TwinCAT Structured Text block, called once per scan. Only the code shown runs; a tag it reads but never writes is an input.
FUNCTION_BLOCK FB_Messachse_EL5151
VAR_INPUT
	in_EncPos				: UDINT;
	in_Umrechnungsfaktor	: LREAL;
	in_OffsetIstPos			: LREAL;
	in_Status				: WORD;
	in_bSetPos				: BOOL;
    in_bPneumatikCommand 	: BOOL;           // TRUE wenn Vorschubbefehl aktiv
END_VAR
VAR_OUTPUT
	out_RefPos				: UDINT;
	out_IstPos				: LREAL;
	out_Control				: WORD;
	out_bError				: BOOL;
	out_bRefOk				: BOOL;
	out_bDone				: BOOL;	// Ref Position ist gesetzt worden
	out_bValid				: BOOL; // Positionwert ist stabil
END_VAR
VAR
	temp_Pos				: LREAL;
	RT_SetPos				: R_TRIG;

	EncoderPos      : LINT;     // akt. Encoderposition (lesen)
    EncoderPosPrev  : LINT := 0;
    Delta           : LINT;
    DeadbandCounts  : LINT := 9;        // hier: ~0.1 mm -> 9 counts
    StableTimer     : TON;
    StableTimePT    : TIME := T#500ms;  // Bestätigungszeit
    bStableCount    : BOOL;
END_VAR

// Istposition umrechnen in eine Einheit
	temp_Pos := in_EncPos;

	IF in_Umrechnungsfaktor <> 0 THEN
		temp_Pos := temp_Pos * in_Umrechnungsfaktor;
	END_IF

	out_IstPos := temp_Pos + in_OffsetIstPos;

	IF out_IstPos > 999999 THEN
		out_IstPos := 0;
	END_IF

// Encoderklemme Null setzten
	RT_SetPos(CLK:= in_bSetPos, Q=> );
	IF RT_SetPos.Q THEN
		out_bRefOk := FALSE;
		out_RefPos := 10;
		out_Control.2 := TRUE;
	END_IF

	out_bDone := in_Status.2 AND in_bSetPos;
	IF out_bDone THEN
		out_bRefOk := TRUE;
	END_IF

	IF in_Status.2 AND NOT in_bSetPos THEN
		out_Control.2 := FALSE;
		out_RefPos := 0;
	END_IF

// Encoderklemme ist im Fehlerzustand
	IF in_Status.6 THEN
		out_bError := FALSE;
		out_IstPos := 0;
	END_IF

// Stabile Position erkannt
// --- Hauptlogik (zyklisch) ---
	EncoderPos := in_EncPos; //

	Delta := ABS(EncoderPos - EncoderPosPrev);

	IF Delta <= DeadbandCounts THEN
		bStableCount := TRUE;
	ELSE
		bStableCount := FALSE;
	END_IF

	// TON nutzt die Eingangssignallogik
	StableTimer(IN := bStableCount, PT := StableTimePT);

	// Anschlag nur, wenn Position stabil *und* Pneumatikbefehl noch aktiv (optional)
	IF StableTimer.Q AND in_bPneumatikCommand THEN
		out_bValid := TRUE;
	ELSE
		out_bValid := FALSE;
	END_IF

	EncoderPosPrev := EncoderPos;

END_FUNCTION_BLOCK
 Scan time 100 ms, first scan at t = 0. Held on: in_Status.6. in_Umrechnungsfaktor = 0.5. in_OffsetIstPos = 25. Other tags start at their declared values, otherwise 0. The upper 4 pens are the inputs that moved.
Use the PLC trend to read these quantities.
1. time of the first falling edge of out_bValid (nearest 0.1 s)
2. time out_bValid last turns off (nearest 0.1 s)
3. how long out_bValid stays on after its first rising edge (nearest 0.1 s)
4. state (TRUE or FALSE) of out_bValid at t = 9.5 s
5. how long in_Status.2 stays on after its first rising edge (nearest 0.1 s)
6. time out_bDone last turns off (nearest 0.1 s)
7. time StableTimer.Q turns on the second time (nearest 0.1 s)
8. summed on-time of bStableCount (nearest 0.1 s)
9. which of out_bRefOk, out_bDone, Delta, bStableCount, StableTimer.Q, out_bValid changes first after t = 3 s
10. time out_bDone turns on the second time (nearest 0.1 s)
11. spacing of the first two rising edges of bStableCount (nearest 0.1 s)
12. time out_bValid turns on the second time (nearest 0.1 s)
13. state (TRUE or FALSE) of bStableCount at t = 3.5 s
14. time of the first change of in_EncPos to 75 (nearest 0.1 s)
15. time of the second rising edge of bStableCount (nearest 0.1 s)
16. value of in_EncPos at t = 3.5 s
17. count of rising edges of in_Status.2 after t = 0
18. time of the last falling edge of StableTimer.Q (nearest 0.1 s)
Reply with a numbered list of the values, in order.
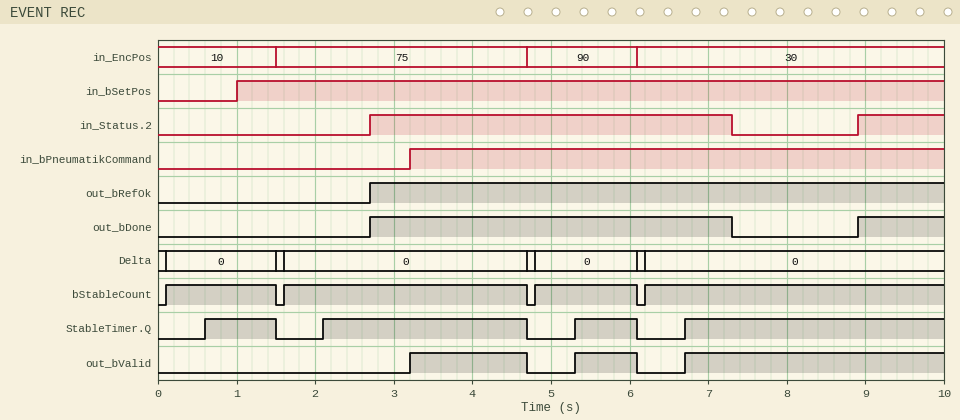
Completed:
1. 4.7 s
2. 6.1 s
3. 1.5 s
4. TRUE
5. 4.6 s
6. 7.3 s
7. 2.1 s
8. 9.6 s
9. out_bValid
10. 8.9 s
11. 1.5 s
12. 5.3 s
13. TRUE
14. 1.5 s
15. 1.6 s
16. 75
17. 2
18. 6.1 s
